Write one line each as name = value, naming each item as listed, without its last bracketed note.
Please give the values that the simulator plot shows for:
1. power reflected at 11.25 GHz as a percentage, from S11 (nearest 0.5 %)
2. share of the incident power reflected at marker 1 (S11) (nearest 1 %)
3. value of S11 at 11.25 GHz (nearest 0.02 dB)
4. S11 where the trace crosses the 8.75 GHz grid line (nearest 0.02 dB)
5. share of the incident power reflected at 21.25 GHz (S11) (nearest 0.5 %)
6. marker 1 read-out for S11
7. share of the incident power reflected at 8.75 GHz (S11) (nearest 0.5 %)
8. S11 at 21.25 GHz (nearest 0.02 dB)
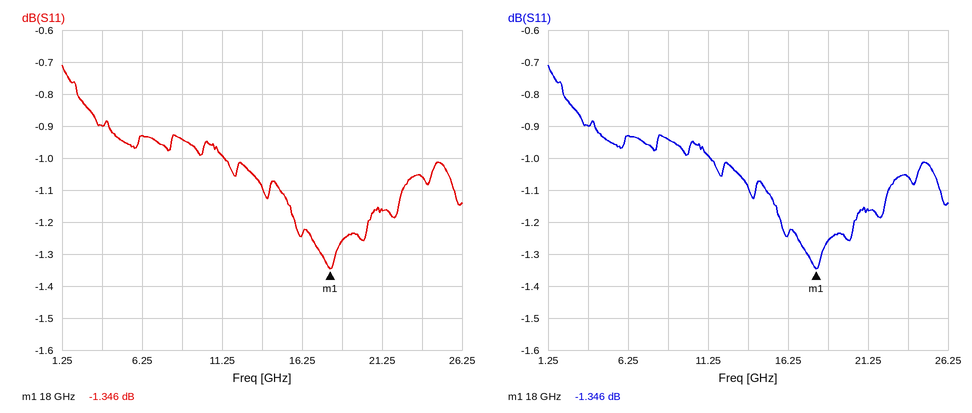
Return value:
power reflected at 11.25 GHz as a percentage, from S11 = 79.5 %
share of the incident power reflected at marker 1 (S11) = 73 %
value of S11 at 11.25 GHz = -1.00 dB
S11 where the trace crosses the 8.75 GHz grid line = -0.94 dB
share of the incident power reflected at 21.25 GHz (S11) = 76.5 %
marker 1 read-out for S11 = -1.346 dB
share of the incident power reflected at 8.75 GHz (S11) = 80.5 %
S11 at 21.25 GHz = -1.16 dB
